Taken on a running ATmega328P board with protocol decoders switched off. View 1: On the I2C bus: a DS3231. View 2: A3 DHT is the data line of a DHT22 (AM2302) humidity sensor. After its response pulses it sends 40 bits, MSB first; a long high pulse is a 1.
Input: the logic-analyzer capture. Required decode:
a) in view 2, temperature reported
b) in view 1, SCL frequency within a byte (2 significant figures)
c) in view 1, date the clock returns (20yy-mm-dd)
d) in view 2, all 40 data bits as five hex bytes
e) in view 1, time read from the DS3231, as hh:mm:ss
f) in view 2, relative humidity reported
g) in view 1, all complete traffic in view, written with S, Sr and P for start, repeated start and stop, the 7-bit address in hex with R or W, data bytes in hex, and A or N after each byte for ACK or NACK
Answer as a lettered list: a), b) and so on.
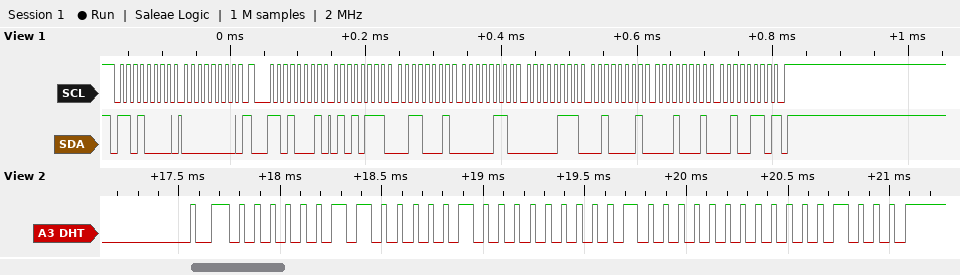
a) 25.6 °C
b) 100 kHz
c) 2026-11-21
d) 03 04 01 00 08
e) 06:31:57
f) 77.2 %
g) S 68W A 00 A Sr 68R A 57 A 31 A 06 A 07 A 21 A 11 A 26 N P
